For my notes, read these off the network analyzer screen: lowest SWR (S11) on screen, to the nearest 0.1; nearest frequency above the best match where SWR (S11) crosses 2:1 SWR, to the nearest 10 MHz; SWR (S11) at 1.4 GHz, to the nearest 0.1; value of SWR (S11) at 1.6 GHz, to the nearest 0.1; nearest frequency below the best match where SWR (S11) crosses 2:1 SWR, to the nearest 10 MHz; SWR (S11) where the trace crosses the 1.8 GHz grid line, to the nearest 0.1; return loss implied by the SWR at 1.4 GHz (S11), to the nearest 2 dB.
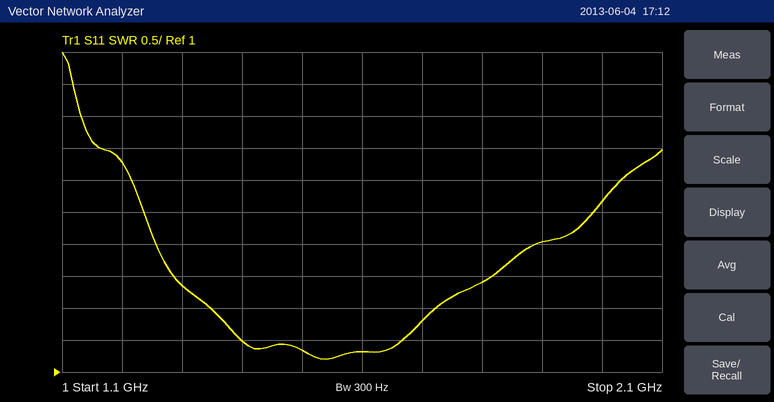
1.2
1.72 GHz
1.5
1.3
1.35 GHz
2.4
14 dB
